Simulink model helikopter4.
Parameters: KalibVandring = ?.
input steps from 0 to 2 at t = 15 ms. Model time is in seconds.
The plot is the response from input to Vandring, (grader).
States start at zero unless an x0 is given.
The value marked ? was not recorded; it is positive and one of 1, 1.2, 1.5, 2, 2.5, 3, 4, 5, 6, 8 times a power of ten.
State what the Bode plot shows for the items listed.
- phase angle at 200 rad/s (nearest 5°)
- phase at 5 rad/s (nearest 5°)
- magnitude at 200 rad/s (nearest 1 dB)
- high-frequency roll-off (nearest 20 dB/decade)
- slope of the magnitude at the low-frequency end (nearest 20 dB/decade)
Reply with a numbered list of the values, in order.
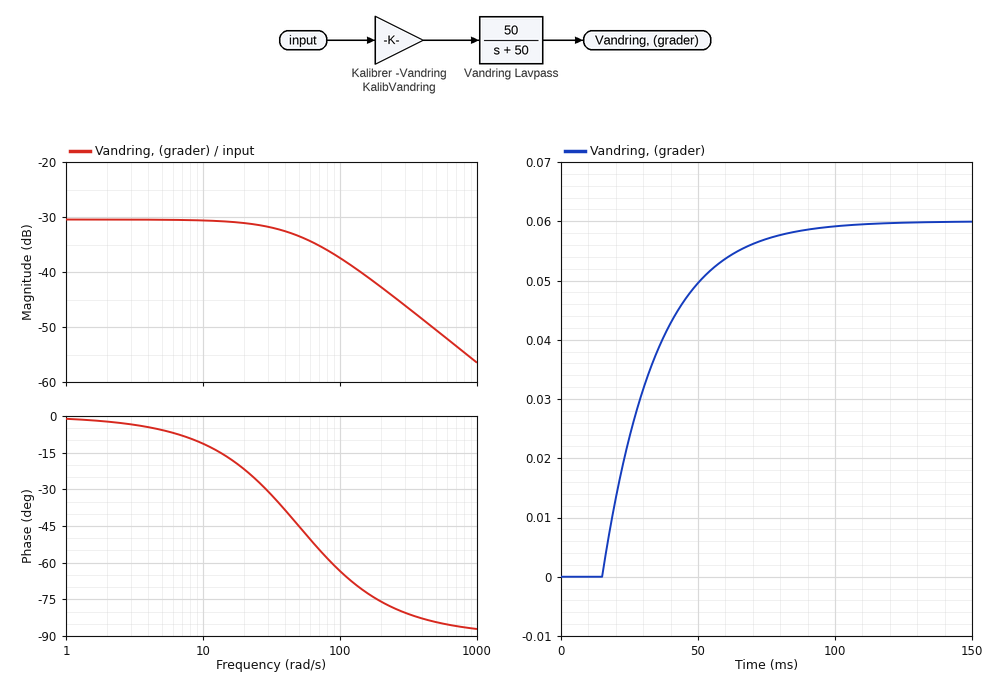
1. -75°
2. -5°
3. -43 dB
4. -20 dB/decade
5. 0 dB/decade
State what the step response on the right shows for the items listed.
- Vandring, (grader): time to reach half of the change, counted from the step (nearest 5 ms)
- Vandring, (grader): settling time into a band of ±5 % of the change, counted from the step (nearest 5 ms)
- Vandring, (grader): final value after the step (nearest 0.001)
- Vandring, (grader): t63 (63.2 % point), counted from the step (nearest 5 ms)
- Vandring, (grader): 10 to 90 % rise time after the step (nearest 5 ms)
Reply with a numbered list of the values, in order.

1. 15 ms
2. 60 ms
3. 0.060
4. 20 ms
5. 45 ms
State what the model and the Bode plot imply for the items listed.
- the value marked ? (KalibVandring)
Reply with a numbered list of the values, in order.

1. 0.03
